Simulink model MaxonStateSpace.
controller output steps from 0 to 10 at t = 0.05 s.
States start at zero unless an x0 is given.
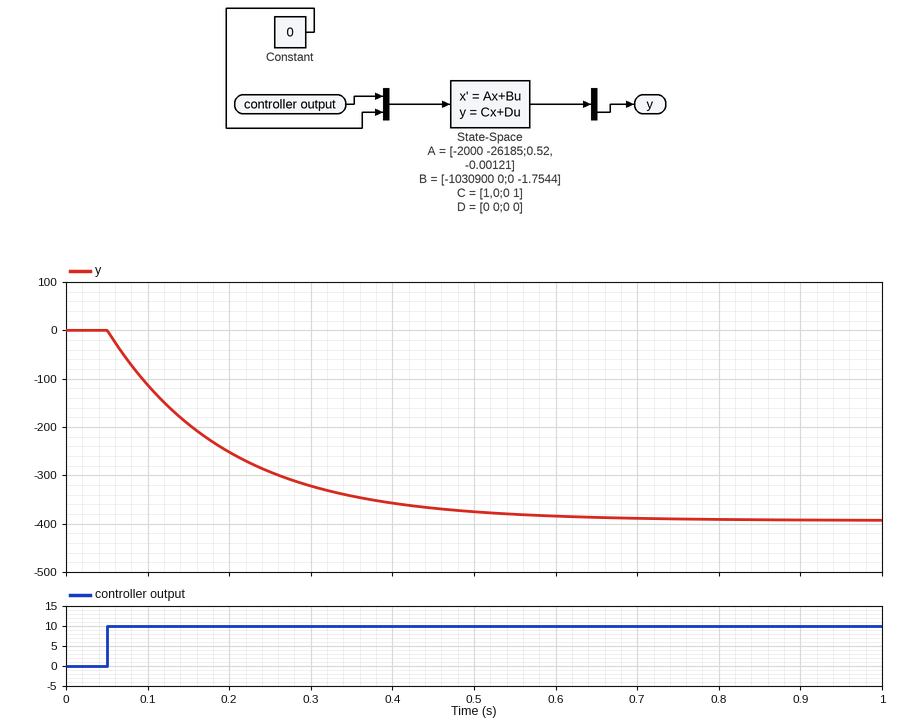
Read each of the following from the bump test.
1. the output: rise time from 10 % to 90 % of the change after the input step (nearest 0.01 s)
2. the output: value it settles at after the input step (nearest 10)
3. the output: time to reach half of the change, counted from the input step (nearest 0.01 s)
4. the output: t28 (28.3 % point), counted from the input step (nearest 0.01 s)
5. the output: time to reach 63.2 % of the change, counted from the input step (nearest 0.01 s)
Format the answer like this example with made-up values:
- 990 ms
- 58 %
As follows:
- 0.32 s
- -390
- 0.10 s
- 0.05 s
- 0.15 s
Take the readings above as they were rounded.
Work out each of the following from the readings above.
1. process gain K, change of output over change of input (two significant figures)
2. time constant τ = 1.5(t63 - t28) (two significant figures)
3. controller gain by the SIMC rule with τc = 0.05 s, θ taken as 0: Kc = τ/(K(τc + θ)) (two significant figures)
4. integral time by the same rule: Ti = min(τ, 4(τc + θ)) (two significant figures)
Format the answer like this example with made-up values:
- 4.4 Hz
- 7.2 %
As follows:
- -39
- 0.15 s
- -0.077
- 0.15 s
